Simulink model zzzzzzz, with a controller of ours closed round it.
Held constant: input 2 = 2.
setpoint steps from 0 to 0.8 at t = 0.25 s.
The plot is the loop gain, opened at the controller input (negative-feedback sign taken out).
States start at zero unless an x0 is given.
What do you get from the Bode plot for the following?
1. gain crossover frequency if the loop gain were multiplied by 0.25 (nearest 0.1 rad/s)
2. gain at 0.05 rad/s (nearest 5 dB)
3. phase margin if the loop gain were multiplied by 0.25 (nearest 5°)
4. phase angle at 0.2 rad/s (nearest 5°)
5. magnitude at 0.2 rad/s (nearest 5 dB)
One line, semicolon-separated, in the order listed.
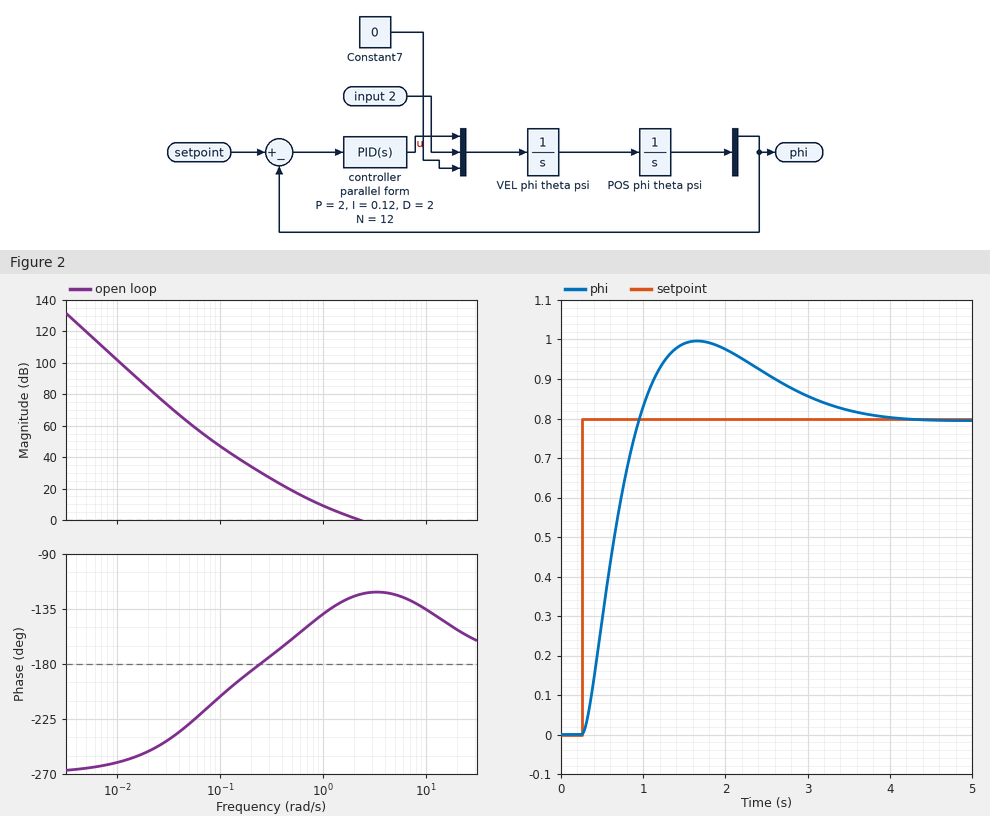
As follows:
0.8 rad/s; 60 dB; 35°; -185°; 35 dB
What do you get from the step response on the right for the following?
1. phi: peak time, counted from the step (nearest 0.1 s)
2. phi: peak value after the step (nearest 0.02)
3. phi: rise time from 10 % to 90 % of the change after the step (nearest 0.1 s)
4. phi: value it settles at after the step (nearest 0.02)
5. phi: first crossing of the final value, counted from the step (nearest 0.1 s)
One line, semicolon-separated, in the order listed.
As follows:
1.4 s; 1.00; 0.5 s; 0.80; 0.7 s
